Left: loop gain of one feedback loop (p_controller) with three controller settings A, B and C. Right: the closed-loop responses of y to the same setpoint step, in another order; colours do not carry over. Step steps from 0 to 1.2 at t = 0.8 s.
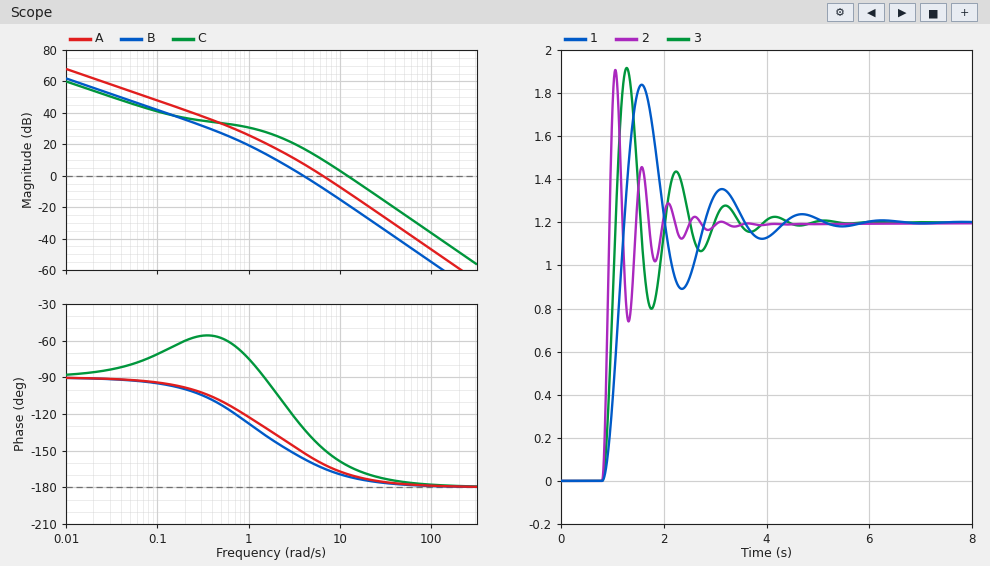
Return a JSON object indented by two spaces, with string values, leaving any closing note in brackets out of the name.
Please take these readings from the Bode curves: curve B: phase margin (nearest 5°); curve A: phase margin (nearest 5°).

{
  "curve B: phase margin": "25°",
  "curve A: phase margin": "20°"
}
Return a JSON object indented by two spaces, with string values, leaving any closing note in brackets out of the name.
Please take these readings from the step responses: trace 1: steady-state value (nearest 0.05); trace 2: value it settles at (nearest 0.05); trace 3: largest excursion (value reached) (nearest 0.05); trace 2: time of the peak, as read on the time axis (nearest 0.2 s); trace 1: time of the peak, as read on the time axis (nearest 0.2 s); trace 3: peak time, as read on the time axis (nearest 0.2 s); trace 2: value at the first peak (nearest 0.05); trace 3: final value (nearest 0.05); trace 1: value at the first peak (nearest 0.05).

{
  "trace 1: steady-state value": "1.20",
  "trace 2: value it settles at": "1.20",
  "trace 3: largest excursion (value reached)": "1.90",
  "trace 2: time of the peak, as read on the time axis": "1.0 s",
  "trace 1: time of the peak, as read on the time axis": "1.6 s",
  "trace 3: peak time, as read on the time axis": "1.2 s",
  "trace 2: value at the first peak": "1.90",
  "trace 3: final value": "1.20",
  "trace 1: value at the first peak": "1.85"
}
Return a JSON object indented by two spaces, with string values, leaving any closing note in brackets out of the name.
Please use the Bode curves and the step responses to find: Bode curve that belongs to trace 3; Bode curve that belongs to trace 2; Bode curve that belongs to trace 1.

{
  "Bode curve that belongs to trace 3": "A",
  "Bode curve that belongs to trace 2": "C",
  "Bode curve that belongs to trace 1": "B"
}
